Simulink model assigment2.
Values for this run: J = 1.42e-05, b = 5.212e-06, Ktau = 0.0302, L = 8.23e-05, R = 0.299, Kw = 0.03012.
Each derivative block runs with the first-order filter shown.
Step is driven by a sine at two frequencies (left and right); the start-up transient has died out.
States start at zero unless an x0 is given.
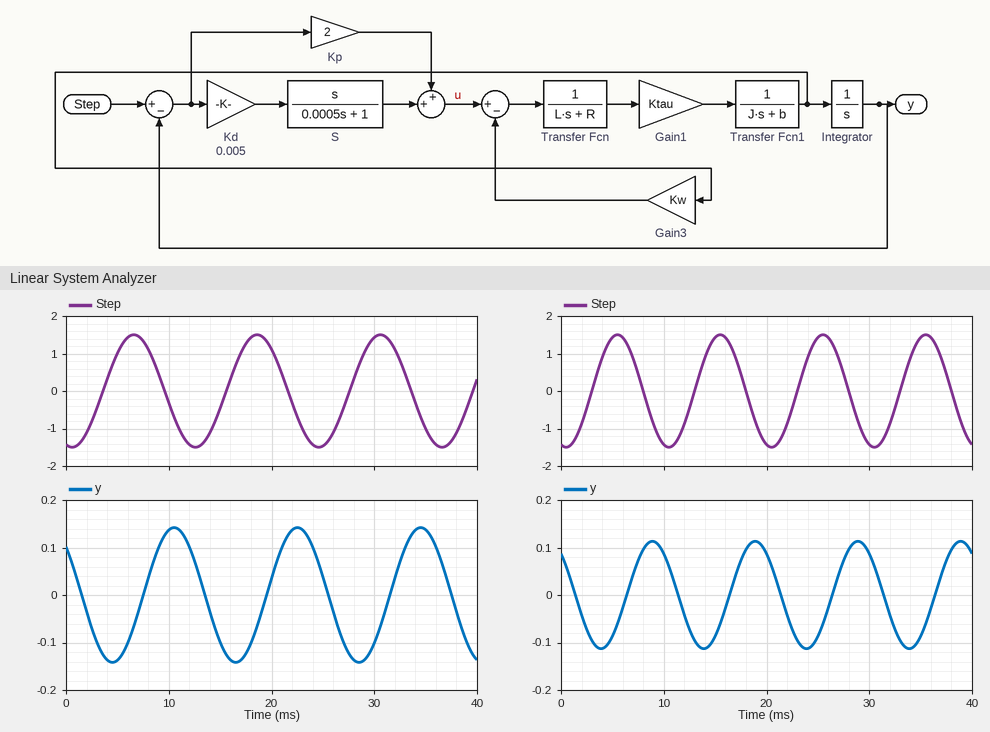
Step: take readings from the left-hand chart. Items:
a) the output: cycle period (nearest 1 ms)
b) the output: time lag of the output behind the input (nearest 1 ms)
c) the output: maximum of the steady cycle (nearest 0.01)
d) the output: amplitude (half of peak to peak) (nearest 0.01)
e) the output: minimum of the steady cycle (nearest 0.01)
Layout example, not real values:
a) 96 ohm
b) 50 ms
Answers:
a) 12 ms
b) 4 ms
c) 0.14
d) 0.14
e) -0.14
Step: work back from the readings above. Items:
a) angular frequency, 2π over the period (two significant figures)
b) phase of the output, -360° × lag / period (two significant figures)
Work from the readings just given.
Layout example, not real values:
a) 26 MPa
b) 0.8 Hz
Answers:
a) 0.52 rad/ms
b) -120°
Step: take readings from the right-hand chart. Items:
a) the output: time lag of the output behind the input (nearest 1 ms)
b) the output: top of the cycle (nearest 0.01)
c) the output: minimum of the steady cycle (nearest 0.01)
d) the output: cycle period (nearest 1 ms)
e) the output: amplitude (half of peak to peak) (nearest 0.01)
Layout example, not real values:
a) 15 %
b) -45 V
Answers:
a) 3 ms
b) 0.11
c) -0.11
d) 10 ms
e) 0.11
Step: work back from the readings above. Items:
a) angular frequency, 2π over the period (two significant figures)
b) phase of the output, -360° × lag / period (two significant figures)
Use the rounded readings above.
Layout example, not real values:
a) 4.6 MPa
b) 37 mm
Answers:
a) 0.63 rad/ms
b) -110°
